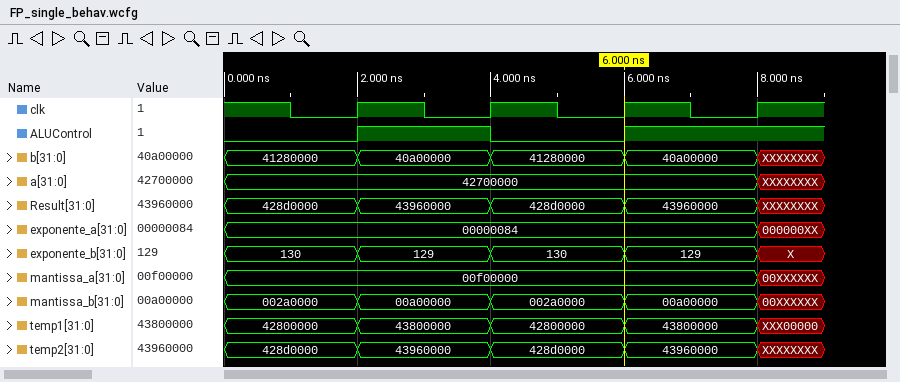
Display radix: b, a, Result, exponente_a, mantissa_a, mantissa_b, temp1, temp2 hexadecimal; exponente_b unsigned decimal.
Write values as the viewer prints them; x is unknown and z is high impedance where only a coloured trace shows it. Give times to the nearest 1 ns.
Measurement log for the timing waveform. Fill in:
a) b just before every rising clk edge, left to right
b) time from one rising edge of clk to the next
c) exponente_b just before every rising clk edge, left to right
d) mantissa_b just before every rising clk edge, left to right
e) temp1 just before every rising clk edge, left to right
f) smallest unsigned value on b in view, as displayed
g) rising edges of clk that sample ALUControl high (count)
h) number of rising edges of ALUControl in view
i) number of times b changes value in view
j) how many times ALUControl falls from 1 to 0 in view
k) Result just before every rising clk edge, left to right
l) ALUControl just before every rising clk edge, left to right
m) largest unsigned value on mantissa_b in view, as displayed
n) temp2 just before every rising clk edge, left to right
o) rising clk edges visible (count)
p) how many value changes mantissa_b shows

41280000, 40a00000, 41280000, 40a00000
2 ns
130, 129, 130, 129
002a0000, 00a00000, 002a0000, 00a00000
42800000, 43800000, 42800000, 43800000
40a00000
2
2
4
1
428d0000, 43960000, 428d0000, 43960000
0 1 0 1
00a00000
428d0000, 43960000, 428d0000, 43960000
4
4
